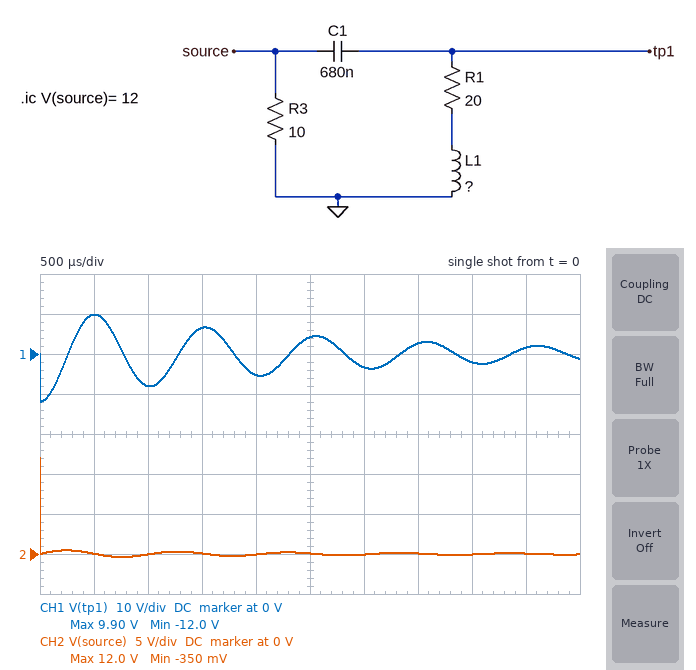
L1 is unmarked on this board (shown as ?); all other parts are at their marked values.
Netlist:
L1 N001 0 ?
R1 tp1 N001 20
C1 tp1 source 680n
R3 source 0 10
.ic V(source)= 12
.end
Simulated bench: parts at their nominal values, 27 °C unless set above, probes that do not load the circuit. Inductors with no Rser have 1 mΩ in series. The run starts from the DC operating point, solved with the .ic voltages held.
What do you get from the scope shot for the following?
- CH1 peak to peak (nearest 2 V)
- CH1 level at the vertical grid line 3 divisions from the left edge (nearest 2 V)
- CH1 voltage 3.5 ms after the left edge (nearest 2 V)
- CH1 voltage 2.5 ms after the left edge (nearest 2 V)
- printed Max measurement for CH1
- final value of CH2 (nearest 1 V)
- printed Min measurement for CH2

22 V
6 V
2 V
4 V
9.90 V
0 V
-350 mV
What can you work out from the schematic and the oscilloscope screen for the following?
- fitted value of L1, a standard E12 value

39 mH
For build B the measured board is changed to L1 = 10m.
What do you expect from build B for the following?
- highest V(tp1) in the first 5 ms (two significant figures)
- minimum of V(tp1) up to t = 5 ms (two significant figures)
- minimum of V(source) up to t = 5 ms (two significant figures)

8.1 V
-12 V
-560 mV
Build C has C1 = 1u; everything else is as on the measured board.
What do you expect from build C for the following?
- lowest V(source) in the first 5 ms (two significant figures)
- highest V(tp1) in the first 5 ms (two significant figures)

-430 mV
9.5 V
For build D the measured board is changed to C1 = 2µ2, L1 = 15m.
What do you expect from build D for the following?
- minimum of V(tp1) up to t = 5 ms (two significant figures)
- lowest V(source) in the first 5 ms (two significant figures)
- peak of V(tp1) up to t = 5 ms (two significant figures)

-12 V
-630 mV
6.8 V
